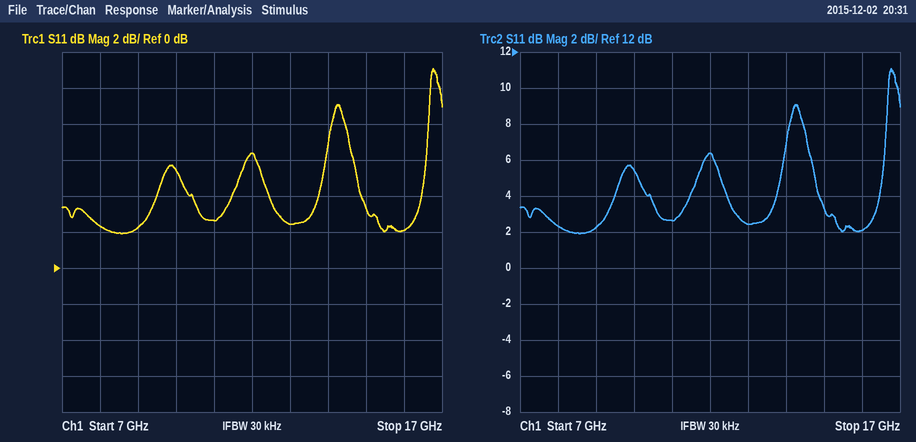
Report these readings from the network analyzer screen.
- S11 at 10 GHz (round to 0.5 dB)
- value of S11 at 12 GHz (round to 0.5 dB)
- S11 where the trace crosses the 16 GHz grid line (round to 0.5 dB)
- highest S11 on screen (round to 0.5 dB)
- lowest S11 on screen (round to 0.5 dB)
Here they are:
5.5 dB
6.5 dB
2.0 dB
11.0 dB
2.0 dB
